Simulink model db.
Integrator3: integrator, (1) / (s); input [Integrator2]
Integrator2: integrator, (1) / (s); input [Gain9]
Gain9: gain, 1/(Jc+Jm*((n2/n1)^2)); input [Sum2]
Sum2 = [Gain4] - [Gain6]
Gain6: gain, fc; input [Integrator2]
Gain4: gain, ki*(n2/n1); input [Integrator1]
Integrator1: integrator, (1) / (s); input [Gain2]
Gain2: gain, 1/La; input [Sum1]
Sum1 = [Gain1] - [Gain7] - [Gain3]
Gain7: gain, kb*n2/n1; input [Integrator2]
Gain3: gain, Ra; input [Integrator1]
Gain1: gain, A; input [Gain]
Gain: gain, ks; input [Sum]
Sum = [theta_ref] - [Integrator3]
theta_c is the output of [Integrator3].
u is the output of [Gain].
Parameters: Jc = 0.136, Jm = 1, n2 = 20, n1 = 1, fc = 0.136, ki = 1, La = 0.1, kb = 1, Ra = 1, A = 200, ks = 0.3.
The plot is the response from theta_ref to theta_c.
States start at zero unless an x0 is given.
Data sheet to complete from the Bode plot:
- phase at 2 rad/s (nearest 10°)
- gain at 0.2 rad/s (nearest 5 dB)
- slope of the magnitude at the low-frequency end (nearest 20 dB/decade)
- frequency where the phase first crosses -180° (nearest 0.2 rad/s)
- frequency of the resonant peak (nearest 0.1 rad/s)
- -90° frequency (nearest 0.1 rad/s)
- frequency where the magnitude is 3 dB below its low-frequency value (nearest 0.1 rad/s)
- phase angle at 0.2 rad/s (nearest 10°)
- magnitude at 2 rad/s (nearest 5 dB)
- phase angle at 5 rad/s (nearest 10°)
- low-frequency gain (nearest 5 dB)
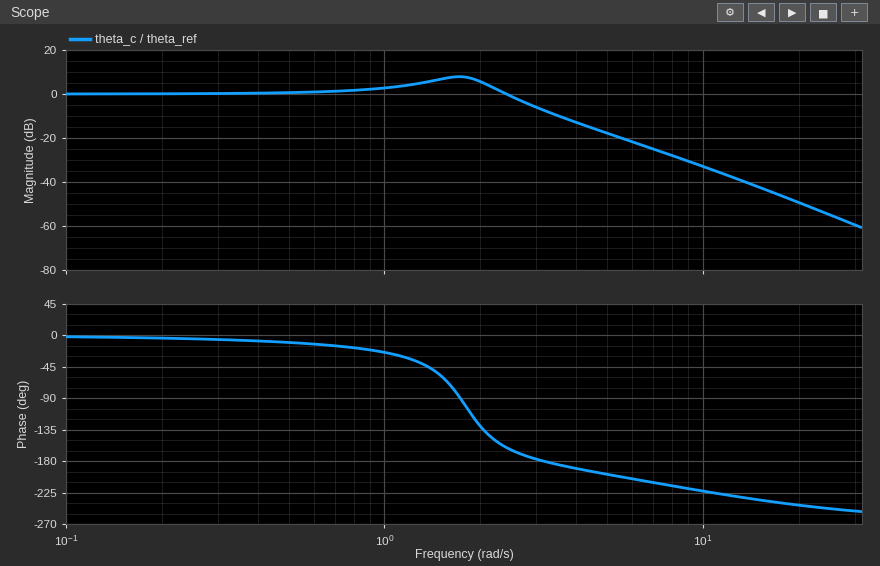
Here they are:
-130°
0 dB
0 dB/decade
3.2 rad/s
1.7 rad/s
1.7 rad/s
2.7 rad/s
0°
5 dB
-200°
0 dB
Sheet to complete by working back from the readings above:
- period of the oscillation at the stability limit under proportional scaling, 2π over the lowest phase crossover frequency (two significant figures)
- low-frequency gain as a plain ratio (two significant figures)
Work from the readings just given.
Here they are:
2.0 s
1.0
